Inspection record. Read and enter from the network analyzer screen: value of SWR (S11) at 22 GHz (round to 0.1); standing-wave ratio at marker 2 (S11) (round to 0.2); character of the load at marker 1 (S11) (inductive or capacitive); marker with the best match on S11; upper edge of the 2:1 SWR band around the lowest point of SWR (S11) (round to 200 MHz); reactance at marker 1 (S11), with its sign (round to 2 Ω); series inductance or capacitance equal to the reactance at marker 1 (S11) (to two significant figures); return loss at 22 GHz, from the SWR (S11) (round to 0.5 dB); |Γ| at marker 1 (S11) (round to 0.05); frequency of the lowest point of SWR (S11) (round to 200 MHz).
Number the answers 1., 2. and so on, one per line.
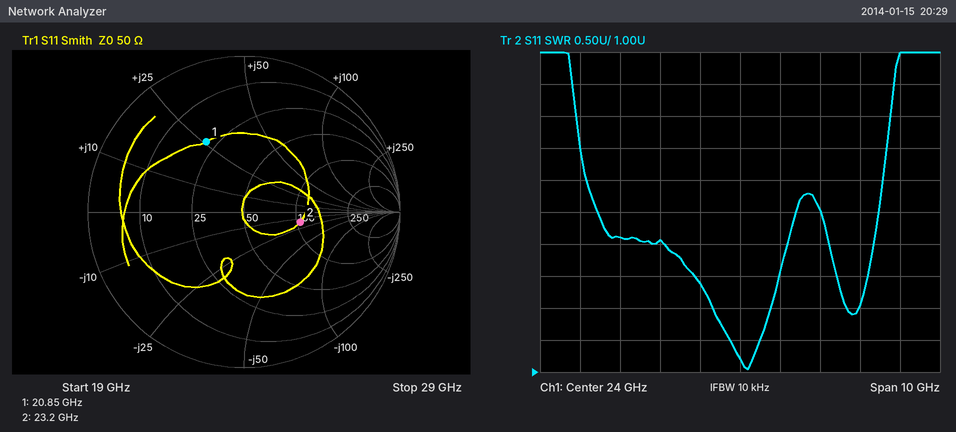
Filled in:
1. 3.1
2. 2.2
3. inductive
4. marker 2
5. 24.8 GHz
6. +26 Ω
7. 200 pH
8. 6.0 dB
9. 0.50
10. 24.2 GHz
